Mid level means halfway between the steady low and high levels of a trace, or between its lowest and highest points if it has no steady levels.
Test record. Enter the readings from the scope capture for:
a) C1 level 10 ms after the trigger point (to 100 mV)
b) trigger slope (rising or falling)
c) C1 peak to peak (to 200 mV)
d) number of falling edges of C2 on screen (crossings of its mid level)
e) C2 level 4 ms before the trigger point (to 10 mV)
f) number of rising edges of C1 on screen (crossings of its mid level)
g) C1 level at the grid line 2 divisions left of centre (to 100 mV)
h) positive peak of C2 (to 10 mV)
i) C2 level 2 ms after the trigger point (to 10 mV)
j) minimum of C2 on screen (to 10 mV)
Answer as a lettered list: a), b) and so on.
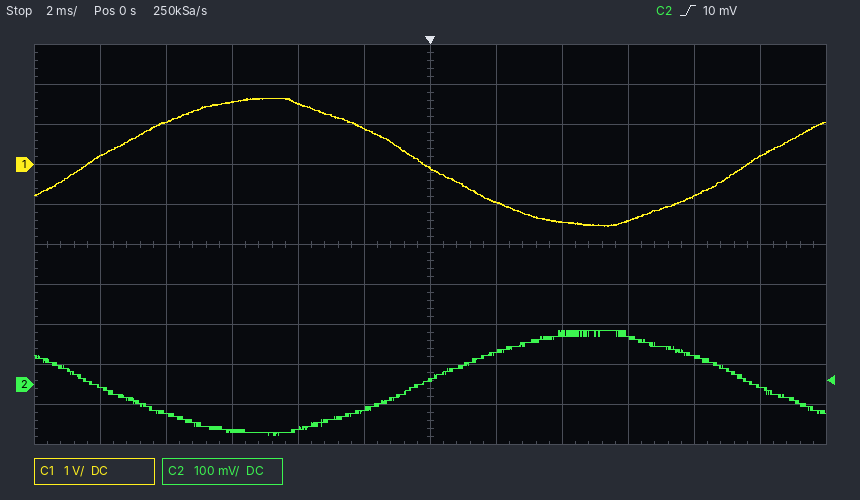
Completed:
a) 200 mV
b) rising
c) 3.2 V
d) 2
e) -110 mV
f) 2
g) 1.5 V
h) 140 mV
i) 80 mV
j) -130 mV
